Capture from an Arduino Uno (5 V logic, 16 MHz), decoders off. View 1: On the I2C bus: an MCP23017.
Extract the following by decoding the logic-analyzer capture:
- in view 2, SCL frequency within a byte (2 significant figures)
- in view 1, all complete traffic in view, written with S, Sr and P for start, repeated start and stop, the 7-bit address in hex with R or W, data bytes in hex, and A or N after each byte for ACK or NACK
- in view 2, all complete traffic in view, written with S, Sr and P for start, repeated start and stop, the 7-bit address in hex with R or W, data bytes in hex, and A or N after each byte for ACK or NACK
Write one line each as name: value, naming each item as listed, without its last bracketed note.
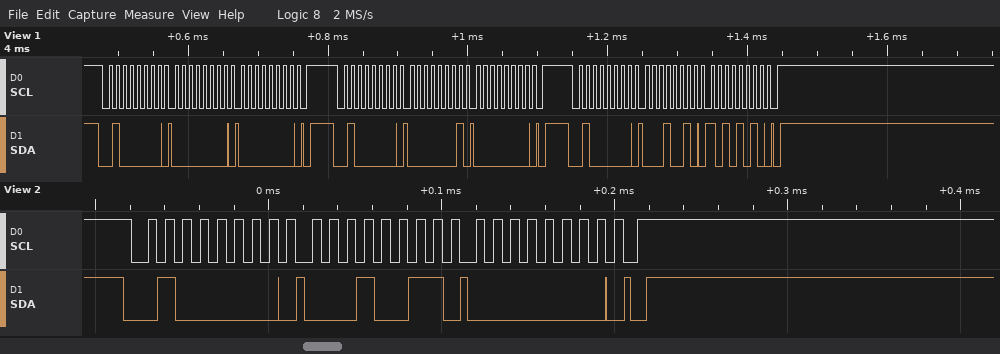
in view 2, SCL frequency within a byte: 100 kHz
in view 1, all complete traffic in view, written with S, Sr and P for start, repeated start and stop, the 7-bit address in hex with R or W, data bytes in hex, and A or N after each byte for ACK or NACK: S 20W A 00 A 00 A P S 20W A 01 A 00 A P S 20W A 12 A AA A P
in view 2, all complete traffic in view, written with S, Sr and P for start, repeated start and stop, the 7-bit address in hex with R or W, data bytes in hex, and A or N after each byte for ACK or NACK: S 20W A 13 A 00 A P
